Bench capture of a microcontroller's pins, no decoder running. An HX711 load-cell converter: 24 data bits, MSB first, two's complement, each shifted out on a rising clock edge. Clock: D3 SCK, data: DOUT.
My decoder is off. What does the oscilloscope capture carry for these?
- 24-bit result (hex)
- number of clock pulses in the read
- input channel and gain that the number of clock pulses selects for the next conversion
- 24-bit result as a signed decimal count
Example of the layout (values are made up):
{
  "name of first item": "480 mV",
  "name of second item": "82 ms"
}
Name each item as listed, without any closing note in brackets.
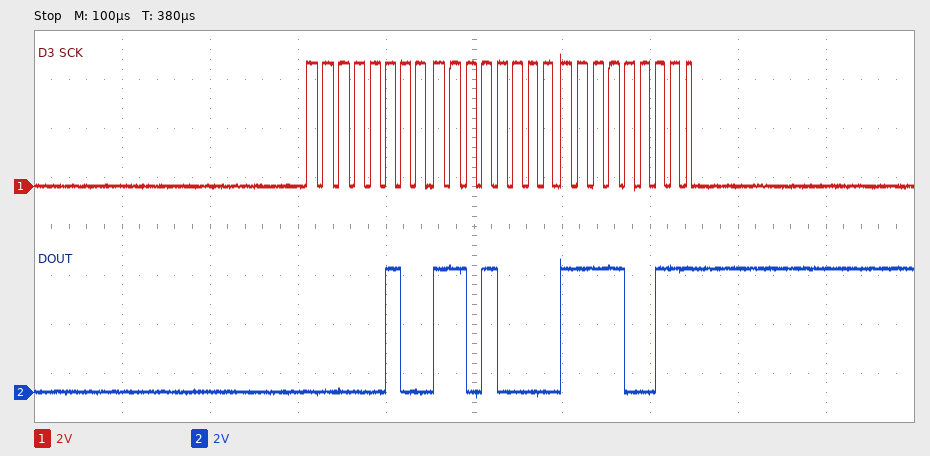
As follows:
{
  "24-bit result": "0x04D0F3",
  "number of clock pulses in the read": "25",
  "input channel and gain that the number of clock pulses selects for the next conversion": "channel A, gain 128",
  "24-bit result as a signed decimal count": "315635"
}
